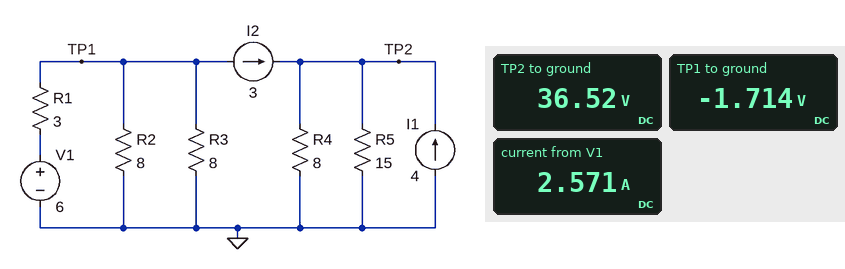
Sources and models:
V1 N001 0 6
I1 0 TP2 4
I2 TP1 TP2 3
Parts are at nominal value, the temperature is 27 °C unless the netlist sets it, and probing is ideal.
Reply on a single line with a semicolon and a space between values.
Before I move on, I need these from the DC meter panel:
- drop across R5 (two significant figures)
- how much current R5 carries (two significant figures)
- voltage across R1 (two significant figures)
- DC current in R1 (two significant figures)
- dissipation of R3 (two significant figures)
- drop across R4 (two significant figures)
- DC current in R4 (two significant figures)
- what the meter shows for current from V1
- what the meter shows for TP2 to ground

37 V; 2.4 A; 7.7 V; 2.6 A; 370 mW; 37 V; 4.6 A; 2.571 A; 36.52 V
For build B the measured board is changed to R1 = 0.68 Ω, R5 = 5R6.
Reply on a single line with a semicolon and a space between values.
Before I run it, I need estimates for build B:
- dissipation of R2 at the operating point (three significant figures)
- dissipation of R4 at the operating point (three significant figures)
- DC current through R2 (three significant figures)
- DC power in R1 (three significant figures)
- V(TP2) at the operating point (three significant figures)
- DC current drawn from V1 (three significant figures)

1.43 W; 66.5 W; 423 mA; 10.1 W; 23.1 V; 3.85 A
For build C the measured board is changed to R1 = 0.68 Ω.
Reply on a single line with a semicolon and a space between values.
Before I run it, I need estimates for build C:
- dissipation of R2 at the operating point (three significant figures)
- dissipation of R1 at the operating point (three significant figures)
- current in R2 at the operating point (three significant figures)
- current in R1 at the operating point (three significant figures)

1.43 W; 10.1 W; 423 mA; 3.85 A
